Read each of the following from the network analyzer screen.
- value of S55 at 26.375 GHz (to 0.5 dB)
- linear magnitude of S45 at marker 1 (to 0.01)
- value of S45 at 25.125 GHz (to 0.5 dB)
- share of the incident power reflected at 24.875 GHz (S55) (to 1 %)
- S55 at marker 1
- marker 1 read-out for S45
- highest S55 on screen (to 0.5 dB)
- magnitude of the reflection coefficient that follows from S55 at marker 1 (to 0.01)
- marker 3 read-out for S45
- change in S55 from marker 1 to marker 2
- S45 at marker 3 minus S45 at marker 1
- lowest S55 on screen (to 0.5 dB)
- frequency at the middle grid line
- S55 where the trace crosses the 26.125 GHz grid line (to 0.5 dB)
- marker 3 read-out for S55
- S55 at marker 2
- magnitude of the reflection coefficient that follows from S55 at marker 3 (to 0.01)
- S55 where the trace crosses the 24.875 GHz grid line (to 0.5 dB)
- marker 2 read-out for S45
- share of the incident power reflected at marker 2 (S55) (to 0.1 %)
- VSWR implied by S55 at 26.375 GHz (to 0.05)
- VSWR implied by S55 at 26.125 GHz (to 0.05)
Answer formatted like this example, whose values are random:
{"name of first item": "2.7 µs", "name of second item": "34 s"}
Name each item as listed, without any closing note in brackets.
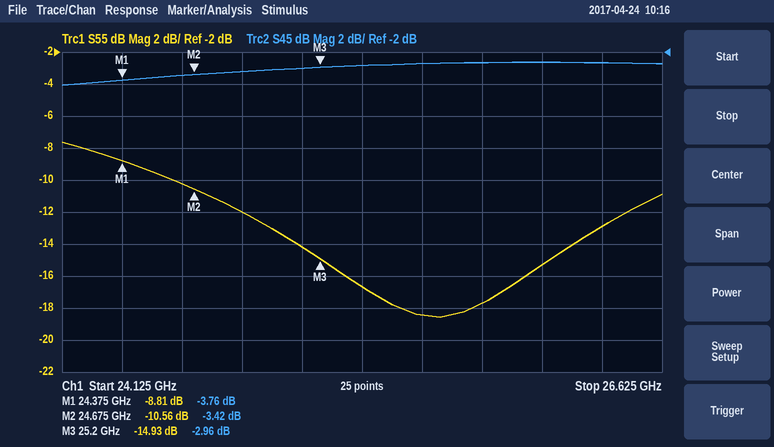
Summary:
{"value of S55 at 26.375 GHz": "-13.0 dB", "linear magnitude of S45 at marker 1": "0.65", "value of S45 at 25.125 GHz": "-3.0 dB", "share of the incident power reflected at 24.875 GHz (S55)": "6 %", "S55 at marker 1": "-8.81 dB", "marker 1 read-out for S45": "-3.76 dB", "highest S55 on screen": "-7.5 dB", "magnitude of the reflection coefficient that follows from S55 at marker 1": "0.36", "marker 3 read-out for S45": "-2.96 dB", "change in S55 from marker 1 to marker 2": "-1.75 dB", "S45 at marker 3 minus S45 at marker 1": "0.80 dB", "lowest S55 on screen": "-18.5 dB", "frequency at the middle grid line": "25.375 GHz", "S55 where the trace crosses the 26.125 GHz grid line": "-15.5 dB", "marker 3 read-out for S55": "-14.93 dB", "S55 at marker 2": "-10.56 dB", "magnitude of the reflection coefficient that follows from S55 at marker 3": "0.18", "S55 where the trace crosses the 24.875 GHz grid line": "-12.0 dB", "marker 2 read-out for S45": "-3.42 dB", "share of the incident power reflected at marker 2 (S55)": "8.8 %", "VSWR implied by S55 at 26.375 GHz": "1.60", "VSWR implied by S55 at 26.125 GHz": "1.40"}
